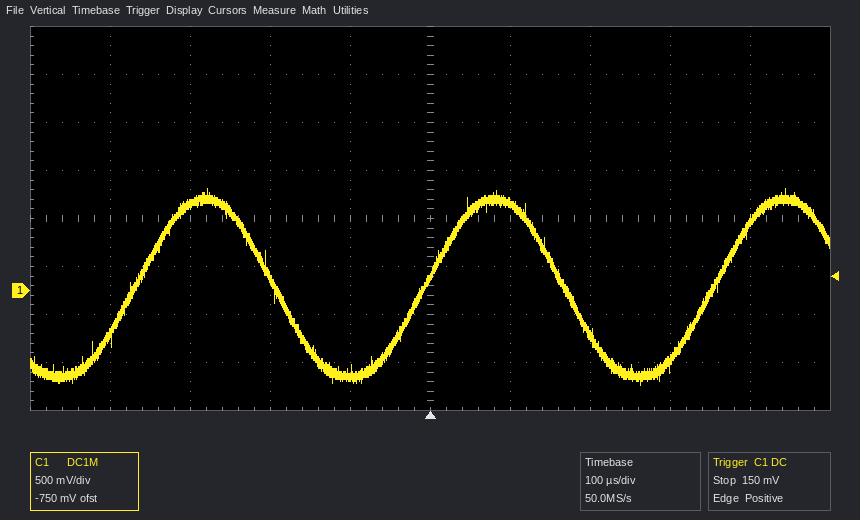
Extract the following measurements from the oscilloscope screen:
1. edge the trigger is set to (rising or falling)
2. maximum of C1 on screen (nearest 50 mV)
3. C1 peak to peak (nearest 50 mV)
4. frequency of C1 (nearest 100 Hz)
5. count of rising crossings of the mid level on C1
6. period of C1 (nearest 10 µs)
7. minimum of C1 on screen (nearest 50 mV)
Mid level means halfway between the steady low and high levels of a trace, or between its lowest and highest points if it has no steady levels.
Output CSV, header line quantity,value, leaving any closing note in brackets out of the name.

quantity,value
edge the trigger is set to,rising
maximum of C1 on screen,1.05 V
C1 peak to peak,2.05 V
frequency of C1,2.8 kHz
count of rising crossings of the mid level on C1,3
period of C1,360 µs
minimum of C1 on screen,-1.00 V
